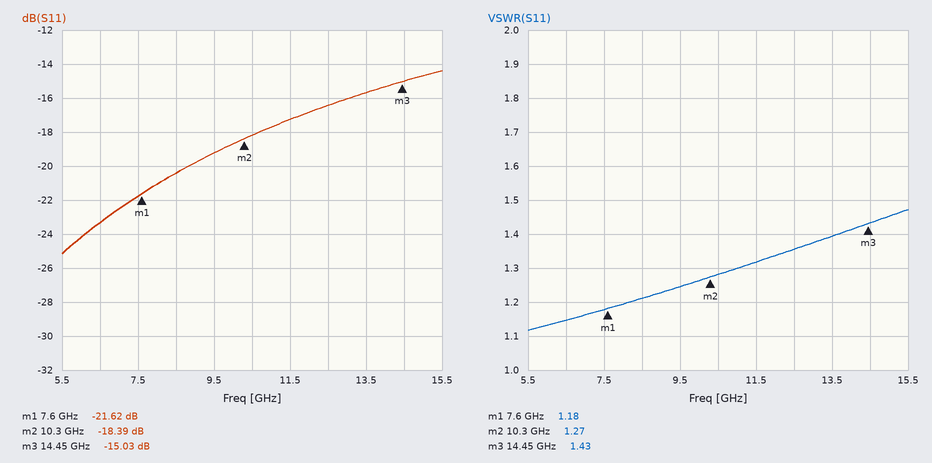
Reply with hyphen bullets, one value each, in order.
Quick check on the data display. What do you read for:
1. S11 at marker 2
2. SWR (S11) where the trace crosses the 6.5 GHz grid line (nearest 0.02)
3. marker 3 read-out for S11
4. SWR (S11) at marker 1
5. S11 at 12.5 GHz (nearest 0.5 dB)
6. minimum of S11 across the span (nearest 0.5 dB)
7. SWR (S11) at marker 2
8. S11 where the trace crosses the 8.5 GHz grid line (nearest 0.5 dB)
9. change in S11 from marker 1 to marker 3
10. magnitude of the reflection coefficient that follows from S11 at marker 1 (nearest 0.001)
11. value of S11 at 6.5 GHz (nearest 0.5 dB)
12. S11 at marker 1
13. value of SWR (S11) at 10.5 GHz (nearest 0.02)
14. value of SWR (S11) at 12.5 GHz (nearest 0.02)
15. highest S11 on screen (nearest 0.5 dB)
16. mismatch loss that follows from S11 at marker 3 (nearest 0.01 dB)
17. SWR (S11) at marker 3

- -18.39 dB
- 1.14
- -15.03 dB
- 1.18
- -16.5 dB
- -25.0 dB
- 1.27
- -20.5 dB
- 6.59 dB
- 0.083
- -23.5 dB
- -21.62 dB
- 1.28
- 1.36
- -14.5 dB
- 0.14 dB
- 1.43
